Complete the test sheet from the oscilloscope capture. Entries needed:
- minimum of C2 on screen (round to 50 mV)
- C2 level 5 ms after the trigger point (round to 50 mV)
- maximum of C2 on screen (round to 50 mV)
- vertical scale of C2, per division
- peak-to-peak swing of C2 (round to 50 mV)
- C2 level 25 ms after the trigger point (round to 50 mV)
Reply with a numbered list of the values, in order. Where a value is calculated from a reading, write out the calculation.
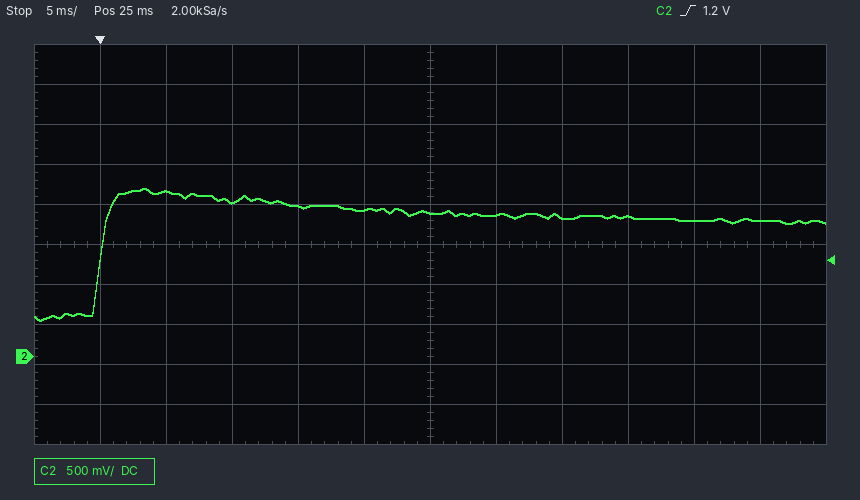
1. 450 mV
2. 2.05 V
3. 2.10 V
4. 500 mV
5. 2.10 V − (450 mV) = 1.65 V
6. 1.80 V
